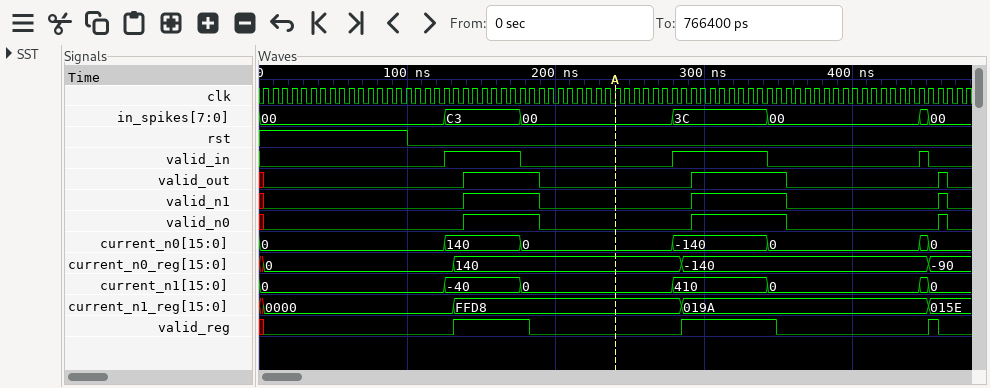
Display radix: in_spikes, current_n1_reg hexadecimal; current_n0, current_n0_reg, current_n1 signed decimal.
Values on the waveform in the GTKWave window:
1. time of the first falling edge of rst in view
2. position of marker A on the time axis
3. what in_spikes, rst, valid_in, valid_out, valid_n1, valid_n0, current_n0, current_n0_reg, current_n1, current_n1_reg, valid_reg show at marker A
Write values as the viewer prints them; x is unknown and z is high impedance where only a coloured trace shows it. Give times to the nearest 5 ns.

100 ns
240 ns
in_spikes=00, rst=0, valid_in=0, valid_out=0, valid_n1=0, valid_n0=0, current_n0=0, current_n0_reg=140, current_n1=0, current_n1_reg=FFD8, valid_reg=0
